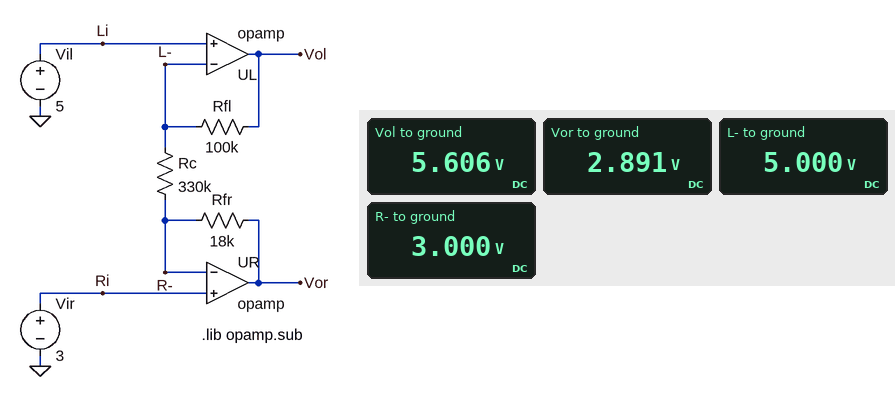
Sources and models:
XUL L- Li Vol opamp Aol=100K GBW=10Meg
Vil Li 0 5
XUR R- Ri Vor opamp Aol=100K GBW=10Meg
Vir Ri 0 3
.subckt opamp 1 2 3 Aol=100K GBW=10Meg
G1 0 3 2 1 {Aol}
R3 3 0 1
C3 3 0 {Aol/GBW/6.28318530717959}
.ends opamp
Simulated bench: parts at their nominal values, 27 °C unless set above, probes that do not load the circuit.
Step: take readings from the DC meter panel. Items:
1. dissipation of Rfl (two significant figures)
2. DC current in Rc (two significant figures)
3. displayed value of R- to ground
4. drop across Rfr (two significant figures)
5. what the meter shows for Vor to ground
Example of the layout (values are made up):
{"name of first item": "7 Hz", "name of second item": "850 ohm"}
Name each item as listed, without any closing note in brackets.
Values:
{"dissipation of Rfl": "3.7 µW", "DC current in Rc": "6.1 µA", "displayed value of R- to ground": "3.000 V", "drop across Rfr": "110 mV", "what the meter shows for Vor to ground": "2.891 V"}
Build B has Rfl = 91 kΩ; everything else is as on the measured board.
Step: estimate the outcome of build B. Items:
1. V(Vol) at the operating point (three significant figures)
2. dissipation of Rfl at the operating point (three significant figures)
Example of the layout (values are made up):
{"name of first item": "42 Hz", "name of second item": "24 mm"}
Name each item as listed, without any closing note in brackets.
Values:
{"V(Vol) at the operating point": "5.55 V", "dissipation of Rfl at the operating point": "3.34 µW"}
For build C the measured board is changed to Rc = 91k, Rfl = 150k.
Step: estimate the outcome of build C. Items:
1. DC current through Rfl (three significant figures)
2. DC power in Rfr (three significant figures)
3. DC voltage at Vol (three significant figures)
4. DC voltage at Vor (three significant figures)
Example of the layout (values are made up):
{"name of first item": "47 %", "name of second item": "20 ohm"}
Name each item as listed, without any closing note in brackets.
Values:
{"DC current through Rfl": "22.0 µA", "DC power in Rfr": "8.69 µW", "DC voltage at Vol": "8.30 V", "DC voltage at Vor": "2.60 V"}
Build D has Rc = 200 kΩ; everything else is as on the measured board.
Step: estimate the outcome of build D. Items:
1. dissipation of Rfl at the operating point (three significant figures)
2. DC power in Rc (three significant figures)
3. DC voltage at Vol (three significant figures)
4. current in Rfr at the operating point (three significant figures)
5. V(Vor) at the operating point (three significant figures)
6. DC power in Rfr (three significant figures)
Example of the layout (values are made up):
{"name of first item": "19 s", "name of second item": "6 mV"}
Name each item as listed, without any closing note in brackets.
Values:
{"dissipation of Rfl at the operating point": "10.0 µW", "DC power in Rc": "20.0 µW", "DC voltage at Vol": "6.00 V", "current in Rfr at the operating point": "10.0 µA", "V(Vor) at the operating point": "2.82 V", "DC power in Rfr": "1.80 µW"}
